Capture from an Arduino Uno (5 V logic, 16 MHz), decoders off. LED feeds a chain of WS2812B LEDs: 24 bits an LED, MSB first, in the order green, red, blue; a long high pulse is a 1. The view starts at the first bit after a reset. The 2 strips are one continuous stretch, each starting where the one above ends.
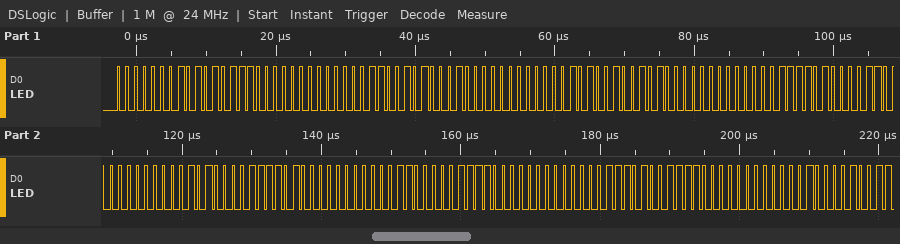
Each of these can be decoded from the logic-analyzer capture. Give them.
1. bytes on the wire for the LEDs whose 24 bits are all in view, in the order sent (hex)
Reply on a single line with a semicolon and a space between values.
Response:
01 57 00 06 51 00 0A 4A 00 0F 43 00 14 3D 00 18 3C 00 1D 3C 00
